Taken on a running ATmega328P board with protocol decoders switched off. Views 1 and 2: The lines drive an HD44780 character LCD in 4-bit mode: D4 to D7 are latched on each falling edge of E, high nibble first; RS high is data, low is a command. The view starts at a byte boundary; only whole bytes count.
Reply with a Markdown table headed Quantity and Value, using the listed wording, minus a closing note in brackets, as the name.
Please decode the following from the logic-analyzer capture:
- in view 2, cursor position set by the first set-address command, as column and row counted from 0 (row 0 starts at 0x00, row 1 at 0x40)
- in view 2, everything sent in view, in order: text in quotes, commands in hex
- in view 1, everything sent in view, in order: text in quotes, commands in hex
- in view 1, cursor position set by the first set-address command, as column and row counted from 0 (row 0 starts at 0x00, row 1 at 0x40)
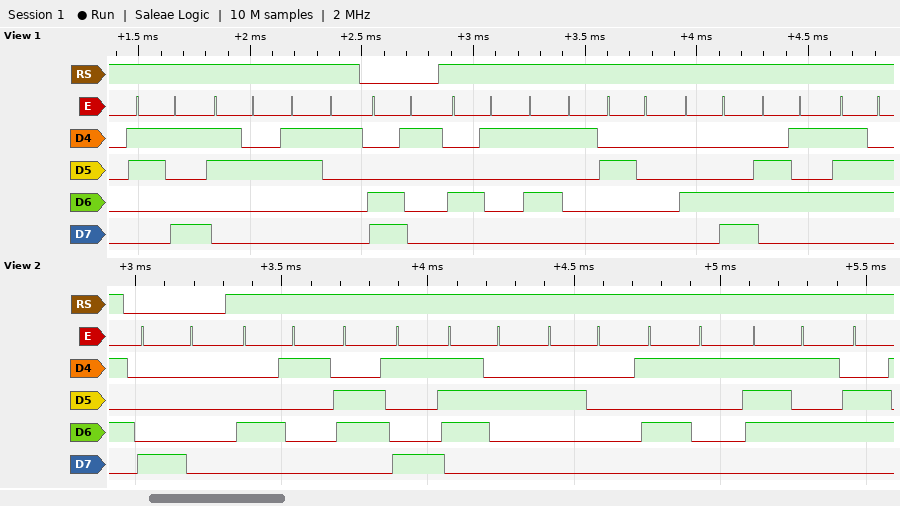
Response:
| Quantity | Value |
|---|---|
| in view 2, cursor position set by the first set-address command, as column and row counted from 0 | column 0, row 0 |
| in view 2, everything sent in view, in order: text in quotes, commands in hex | 0x80 "Air Qu" |
| in view 1, everything sent in view, in order: text in quotes, commands in hex | "921" 0xC1 "AQ Lev" |
| in view 1, cursor position set by the first set-address command, as column and row counted from 0 | column 1, row 1 |
